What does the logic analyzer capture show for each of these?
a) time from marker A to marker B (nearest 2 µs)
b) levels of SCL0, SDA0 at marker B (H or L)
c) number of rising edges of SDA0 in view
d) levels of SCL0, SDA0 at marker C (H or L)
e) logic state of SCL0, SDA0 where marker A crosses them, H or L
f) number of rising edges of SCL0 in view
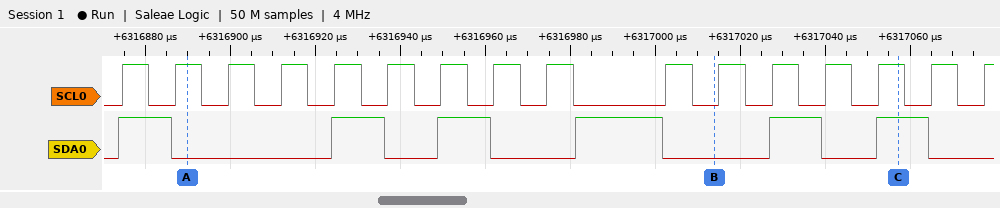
124 µs
SCL0=L, SDA0=L
6
SCL0=H, SDA0=H
SCL0=H, SDA0=L
16
